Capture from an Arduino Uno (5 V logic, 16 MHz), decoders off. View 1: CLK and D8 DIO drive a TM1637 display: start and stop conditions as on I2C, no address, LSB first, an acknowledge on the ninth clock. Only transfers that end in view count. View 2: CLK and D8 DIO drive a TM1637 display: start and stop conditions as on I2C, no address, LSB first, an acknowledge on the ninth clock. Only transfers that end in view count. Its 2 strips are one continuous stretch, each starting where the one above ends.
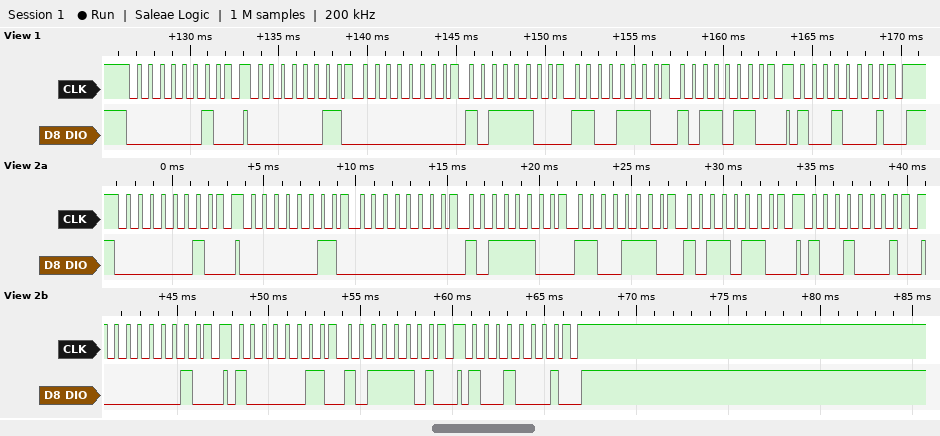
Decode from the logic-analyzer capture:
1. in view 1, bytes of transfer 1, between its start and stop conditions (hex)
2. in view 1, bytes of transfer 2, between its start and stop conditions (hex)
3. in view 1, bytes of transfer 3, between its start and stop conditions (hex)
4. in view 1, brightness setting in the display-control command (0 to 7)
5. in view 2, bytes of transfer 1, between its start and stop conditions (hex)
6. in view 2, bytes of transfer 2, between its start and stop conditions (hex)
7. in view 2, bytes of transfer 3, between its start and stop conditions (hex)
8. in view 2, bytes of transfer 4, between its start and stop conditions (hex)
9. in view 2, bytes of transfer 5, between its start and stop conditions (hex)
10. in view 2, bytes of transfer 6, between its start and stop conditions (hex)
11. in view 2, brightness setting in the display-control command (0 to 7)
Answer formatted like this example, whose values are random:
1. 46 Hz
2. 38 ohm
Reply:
1. 40
2. C0 00 3D 73 6D
3. 89
4. 1
5. 40
6. C0 00 3D 73 6D
7. 89
8. 40
9. C1 BD
10. 89
11. 1
